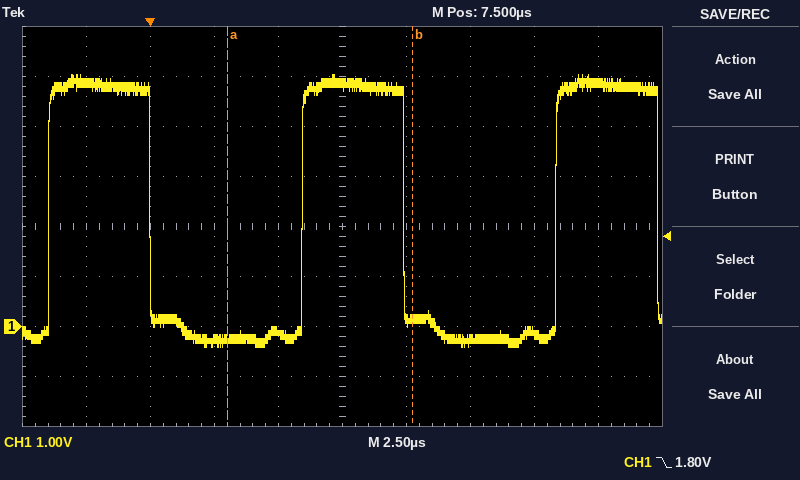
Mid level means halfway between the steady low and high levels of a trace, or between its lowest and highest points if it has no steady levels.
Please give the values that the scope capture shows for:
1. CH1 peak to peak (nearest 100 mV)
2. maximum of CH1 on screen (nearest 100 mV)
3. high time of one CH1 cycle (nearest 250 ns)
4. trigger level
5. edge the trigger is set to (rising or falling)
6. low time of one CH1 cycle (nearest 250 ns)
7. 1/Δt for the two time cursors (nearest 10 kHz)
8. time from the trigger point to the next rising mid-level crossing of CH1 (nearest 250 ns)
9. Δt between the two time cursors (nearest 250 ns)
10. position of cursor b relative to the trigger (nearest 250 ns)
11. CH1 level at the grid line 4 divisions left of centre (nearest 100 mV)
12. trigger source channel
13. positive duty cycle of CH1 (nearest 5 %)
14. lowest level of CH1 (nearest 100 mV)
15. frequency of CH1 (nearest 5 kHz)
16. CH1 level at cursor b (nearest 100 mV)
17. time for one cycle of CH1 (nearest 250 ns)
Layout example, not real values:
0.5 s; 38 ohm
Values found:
5.4 V; 5.0 V; 4.00 µs; 1.80 V; falling; 6.00 µs; 140 kHz; 6.00 µs; 7.25 µs; +10.25 µs; 4.9 V; CH1; 40 %; -400 mV; 100 kHz; 200 mV; 10.00 µs
